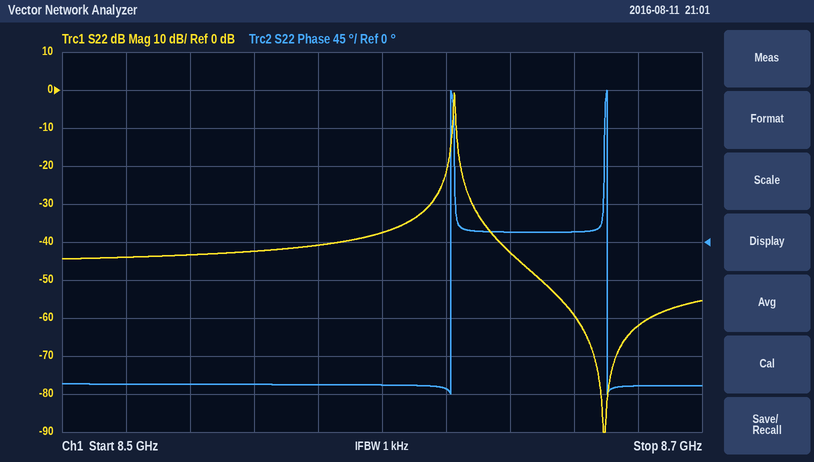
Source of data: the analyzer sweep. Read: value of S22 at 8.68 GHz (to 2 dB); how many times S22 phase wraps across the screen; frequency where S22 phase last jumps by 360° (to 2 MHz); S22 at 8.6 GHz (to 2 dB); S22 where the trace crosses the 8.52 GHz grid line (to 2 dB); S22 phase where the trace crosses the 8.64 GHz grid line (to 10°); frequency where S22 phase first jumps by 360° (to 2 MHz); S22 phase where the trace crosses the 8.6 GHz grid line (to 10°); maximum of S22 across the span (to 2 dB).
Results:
-62 dB
2
8.670 GHz
-38 dB
-44 dB
10°
8.622 GHz
-170°
0 dB
